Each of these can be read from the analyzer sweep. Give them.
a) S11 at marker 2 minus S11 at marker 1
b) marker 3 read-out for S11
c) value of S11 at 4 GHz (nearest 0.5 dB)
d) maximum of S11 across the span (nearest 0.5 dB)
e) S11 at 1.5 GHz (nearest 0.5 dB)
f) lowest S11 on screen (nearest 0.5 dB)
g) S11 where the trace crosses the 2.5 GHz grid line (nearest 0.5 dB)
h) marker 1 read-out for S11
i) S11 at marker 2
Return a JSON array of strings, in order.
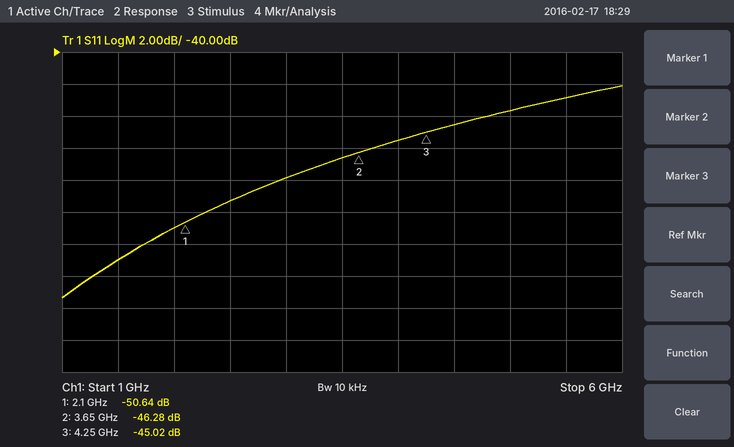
["4.36 dB", "-45.02 dB", "-45.5 dB", "-42.0 dB", "-53.0 dB", "-55.5 dB", "-49.5 dB", "-50.64 dB", "-46.28 dB"]
